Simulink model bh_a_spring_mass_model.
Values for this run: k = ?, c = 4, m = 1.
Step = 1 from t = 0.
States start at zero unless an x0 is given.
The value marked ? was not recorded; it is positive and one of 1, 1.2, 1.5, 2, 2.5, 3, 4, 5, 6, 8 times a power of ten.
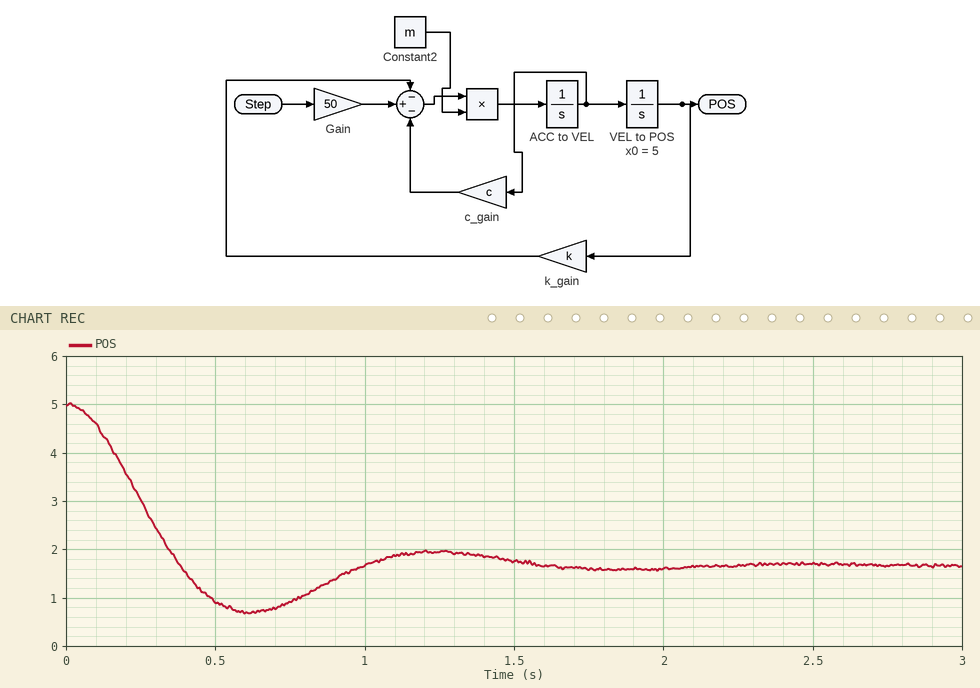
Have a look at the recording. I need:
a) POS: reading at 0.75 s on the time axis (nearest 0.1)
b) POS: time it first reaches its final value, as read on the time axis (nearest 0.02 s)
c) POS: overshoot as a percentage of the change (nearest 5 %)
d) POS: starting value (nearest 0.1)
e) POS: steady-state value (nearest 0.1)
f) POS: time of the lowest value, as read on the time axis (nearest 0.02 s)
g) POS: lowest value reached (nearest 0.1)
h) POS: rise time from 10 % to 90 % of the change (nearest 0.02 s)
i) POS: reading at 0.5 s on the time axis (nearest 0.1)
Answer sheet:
0.9
0.38 s
30 %
5.0
1.7
0.62 s
0.7
0.26 s
0.9
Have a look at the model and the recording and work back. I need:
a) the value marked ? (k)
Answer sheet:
30
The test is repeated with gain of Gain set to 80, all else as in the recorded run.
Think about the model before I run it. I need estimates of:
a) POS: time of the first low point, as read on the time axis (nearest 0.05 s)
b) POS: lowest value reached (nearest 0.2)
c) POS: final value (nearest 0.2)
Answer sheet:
0.60 s
2.0
2.6
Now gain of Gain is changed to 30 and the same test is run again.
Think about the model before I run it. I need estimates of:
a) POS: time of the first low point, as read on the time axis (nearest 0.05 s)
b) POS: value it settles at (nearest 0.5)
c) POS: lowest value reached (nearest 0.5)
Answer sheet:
0.60 s
1.0
0.0
